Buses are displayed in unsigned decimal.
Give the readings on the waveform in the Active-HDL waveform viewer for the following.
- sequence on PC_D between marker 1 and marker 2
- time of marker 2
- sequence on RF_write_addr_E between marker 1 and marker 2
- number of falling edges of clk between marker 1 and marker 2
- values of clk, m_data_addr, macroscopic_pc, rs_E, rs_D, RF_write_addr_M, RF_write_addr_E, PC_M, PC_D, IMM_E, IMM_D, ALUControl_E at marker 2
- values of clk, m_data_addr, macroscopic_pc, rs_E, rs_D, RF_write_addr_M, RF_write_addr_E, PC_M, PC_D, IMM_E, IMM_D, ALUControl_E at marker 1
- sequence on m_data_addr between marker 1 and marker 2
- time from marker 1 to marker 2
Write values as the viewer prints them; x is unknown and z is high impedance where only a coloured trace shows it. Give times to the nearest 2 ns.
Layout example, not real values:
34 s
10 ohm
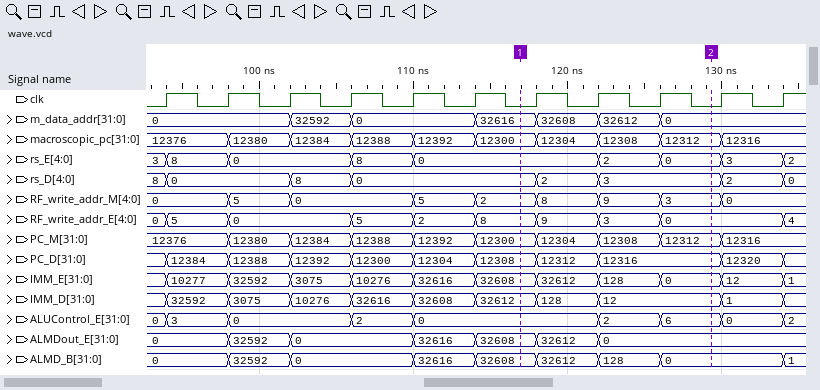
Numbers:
12308, 12312, 12316
130 ns
8, 9, 3, 0
3
clk=0, m_data_addr=0, macroscopic_pc=12312, rs_E=0, rs_D=3, RF_write_addr_M=3, RF_write_addr_E=0, PC_M=12312, PC_D=12316, IMM_E=0, IMM_D=12, ALUControl_E=6
clk=0, m_data_addr=32616, macroscopic_pc=12300, rs_E=0, rs_D=0, RF_write_addr_M=2, RF_write_addr_E=8, PC_M=12300, PC_D=12308, IMM_E=32608, IMM_D=32612, ALUControl_E=0
32616, 32608, 32612, 0
12 ns
